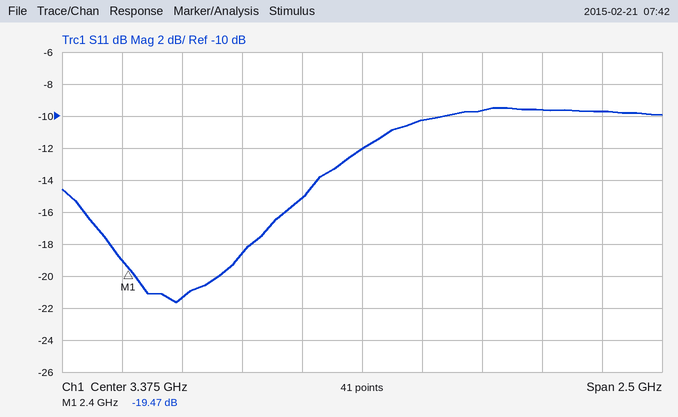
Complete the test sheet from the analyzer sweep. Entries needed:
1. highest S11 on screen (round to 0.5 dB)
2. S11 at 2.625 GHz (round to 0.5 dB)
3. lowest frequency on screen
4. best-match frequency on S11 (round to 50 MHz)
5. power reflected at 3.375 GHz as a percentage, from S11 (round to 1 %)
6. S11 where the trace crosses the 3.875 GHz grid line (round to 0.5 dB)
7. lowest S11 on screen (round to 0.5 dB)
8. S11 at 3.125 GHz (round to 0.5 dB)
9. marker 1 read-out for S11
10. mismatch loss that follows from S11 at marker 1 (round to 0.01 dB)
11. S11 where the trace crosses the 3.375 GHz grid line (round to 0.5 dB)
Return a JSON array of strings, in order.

["-9.5 dB", "-21.5 dB", "2.125 GHz", "2.60 GHz", "6 %", "-9.5 dB", "-21.5 dB", "-15.0 dB", "-19.47 dB", "0.05 dB", "-12.0 dB"]
